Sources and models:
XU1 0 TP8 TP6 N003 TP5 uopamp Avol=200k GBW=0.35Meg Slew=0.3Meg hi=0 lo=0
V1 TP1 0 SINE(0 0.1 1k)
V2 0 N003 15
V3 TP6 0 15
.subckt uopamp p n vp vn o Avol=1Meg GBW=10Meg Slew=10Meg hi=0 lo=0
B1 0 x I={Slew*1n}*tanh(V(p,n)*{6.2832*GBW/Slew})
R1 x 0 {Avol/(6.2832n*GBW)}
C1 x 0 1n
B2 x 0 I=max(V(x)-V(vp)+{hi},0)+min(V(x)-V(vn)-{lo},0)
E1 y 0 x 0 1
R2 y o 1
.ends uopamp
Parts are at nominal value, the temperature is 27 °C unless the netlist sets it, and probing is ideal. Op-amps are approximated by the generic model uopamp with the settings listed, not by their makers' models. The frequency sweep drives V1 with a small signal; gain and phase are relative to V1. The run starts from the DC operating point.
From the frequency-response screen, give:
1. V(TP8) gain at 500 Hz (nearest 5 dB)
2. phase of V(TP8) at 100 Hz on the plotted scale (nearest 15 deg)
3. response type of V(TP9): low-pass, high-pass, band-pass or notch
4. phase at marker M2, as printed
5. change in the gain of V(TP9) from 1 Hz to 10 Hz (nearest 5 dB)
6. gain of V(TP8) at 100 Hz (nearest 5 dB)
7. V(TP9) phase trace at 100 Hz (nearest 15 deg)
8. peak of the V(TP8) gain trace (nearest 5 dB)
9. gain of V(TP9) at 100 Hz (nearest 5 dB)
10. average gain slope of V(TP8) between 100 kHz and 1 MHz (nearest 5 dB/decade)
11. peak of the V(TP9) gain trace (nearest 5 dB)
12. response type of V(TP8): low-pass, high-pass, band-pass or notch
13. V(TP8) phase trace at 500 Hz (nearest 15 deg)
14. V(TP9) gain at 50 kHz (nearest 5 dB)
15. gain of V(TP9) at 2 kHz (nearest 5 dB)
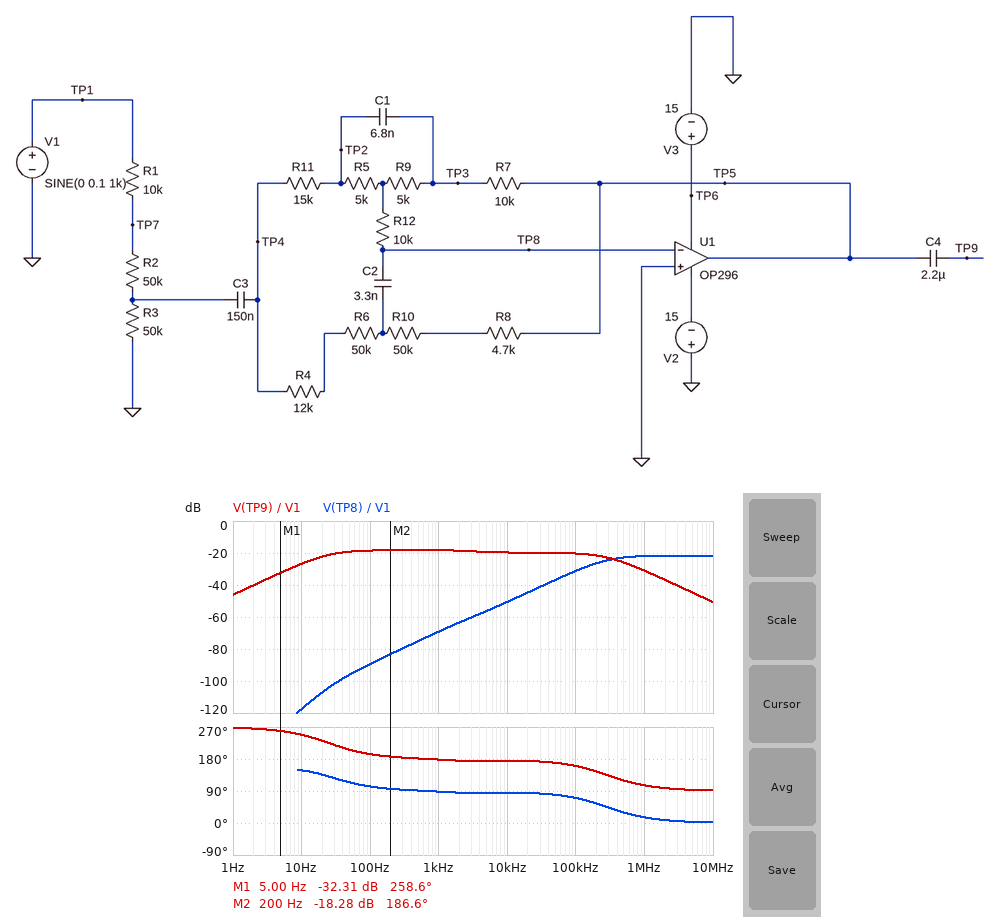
-75 dB
105 deg
band-pass
186.6 deg
20 dB
-90 dB
195 deg
-20 dB
-20 dB
10 dB/decade
-20 dB
high-pass
90 deg
-20 dB
-20 dB
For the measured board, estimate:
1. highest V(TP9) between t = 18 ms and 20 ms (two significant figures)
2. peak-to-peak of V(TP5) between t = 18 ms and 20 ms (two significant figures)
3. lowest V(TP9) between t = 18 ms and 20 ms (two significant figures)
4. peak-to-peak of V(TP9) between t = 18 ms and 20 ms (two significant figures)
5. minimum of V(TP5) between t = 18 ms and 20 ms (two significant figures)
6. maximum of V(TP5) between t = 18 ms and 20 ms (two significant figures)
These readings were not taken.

12 mV
24 mV
-12 mV
24 mV
-12 mV
12 mV
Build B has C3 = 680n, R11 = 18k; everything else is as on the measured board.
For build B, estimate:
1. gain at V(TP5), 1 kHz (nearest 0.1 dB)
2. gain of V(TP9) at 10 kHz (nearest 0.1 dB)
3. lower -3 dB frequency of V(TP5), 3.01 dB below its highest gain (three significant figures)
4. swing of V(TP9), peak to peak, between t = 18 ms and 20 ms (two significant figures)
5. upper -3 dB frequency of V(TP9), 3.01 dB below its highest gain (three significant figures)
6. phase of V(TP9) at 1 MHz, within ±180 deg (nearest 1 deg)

-18.6 dB
-19.8 dB
5.40 Hz
23 mV
198 kHz
106 deg
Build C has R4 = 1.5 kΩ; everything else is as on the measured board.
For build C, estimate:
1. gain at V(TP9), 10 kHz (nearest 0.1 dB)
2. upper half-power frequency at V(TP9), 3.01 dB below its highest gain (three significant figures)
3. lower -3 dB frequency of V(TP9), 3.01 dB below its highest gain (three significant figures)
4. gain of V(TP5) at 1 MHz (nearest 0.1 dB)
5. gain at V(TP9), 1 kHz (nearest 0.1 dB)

-19.3 dB
198 kHz
26.1 Hz
-30.7 dB
-18.2 dB
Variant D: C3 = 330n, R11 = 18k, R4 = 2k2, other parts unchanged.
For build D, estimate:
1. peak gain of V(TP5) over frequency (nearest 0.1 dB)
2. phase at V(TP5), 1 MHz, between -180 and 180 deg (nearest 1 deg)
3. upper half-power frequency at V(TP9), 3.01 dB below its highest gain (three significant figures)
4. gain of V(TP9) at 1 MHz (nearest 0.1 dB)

-18.5 dB
106 deg
214 kHz
-30.8 dB
